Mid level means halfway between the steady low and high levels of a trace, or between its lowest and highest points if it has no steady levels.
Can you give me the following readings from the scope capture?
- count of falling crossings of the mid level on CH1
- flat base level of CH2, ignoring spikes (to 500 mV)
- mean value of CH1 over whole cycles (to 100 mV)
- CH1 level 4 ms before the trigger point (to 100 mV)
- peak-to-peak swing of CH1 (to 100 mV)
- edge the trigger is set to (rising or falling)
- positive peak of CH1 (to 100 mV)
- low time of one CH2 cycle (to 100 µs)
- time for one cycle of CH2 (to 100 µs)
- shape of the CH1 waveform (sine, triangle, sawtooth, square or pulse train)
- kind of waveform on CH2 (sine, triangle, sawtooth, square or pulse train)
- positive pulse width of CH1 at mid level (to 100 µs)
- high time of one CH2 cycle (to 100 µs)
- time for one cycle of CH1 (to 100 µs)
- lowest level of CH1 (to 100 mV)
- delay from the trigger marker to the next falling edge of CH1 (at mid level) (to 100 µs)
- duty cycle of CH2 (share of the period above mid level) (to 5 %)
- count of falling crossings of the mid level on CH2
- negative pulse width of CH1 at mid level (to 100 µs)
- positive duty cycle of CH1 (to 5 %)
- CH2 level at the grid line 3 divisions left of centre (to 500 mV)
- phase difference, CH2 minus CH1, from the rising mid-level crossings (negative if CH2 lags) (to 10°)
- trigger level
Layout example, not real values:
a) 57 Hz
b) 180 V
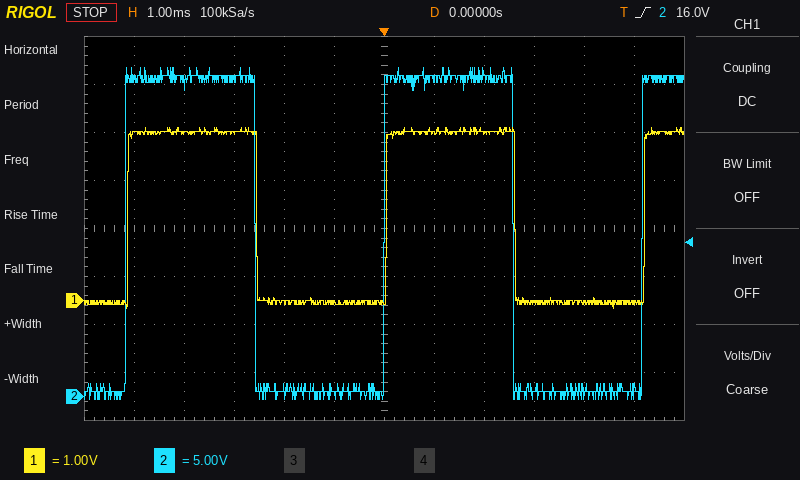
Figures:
a) 2
b) 500 mV
c) 1.7 V
d) 3.5 V
e) 3.8 V
f) rising
g) 3.6 V
h) 2.6 ms
i) 5.2 ms
j) square
k) square
l) 2.6 ms
m) 2.6 ms
n) 5.2 ms
o) -200 mV
p) 2.6 ms
q) 50 %
r) 2
s) 2.6 ms
t) 50 %
u) 33.0 V
v) 0°
w) 16.0 V
